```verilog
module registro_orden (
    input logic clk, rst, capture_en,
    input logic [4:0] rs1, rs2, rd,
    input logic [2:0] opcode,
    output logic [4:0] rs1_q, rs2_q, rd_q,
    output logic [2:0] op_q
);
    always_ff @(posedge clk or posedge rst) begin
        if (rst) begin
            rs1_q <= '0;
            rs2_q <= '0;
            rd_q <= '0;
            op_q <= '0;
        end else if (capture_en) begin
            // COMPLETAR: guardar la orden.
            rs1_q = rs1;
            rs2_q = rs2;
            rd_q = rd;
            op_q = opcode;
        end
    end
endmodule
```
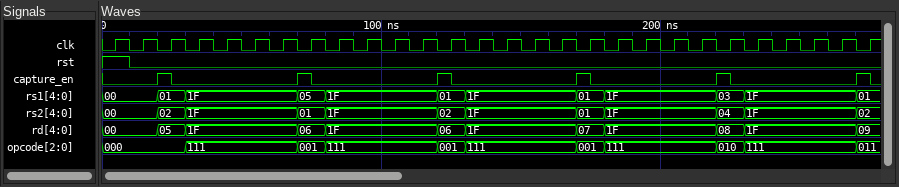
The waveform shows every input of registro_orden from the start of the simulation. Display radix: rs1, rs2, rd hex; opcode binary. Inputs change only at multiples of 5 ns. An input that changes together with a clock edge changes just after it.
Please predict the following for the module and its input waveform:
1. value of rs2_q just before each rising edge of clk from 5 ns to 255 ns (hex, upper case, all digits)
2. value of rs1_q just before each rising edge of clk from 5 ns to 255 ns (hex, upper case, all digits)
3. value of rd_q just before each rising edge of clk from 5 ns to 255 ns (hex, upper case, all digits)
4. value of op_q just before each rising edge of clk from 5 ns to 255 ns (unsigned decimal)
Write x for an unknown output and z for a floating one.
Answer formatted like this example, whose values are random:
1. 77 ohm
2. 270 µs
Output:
1. 00, 00, 00, 02, 02, 02, 02, 02, 01, 01, 01, 01, 01, 02, 02, 02, 02, 02, 01, 01, 01, 01, 01, 04, 04, 04
2. 00, 00, 00, 01, 01, 01, 01, 01, 05, 05, 05, 05, 05, 01, 01, 01, 01, 01, 01, 01, 01, 01, 01, 03, 03, 03
3. 00, 00, 00, 05, 05, 05, 05, 05, 06, 06, 06, 06, 06, 06, 06, 06, 06, 06, 07, 07, 07, 07, 07, 08, 08, 08
4. 0, 0, 0, 0, 0, 0, 0, 0, 1, 1, 1, 1, 1, 1, 1, 1, 1, 1, 1, 1, 1, 1, 1, 2, 2, 2
